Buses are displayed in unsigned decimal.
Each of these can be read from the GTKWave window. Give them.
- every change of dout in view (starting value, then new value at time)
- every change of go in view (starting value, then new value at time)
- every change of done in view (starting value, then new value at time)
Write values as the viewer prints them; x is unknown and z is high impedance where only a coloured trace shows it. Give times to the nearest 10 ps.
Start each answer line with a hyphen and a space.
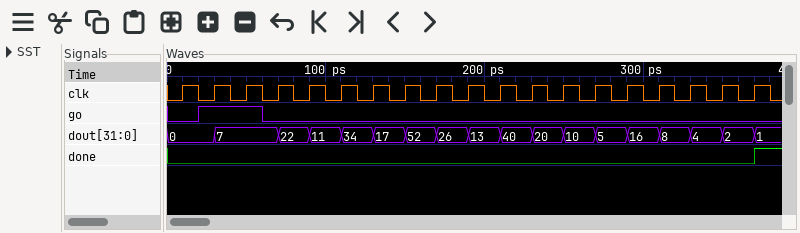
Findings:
- 0, 7 at 30 ps, 22 at 70 ps, 11 at 90 ps, 34 at 110 ps, 17 at 130 ps, 52 at 150 ps, 26 at 170 ps, 13 at 190 ps, 40 at 210 ps, 20 at 230 ps, 10 at 250 ps, 5 at 270 ps, 16 at 290 ps, 8 at 310 ps, 4 at 330 ps, 2 at 350 ps, 1 at 370 ps
- 0, 1 at 20 ps, 0 at 60 ps
- 0, 1 at 370 ps
